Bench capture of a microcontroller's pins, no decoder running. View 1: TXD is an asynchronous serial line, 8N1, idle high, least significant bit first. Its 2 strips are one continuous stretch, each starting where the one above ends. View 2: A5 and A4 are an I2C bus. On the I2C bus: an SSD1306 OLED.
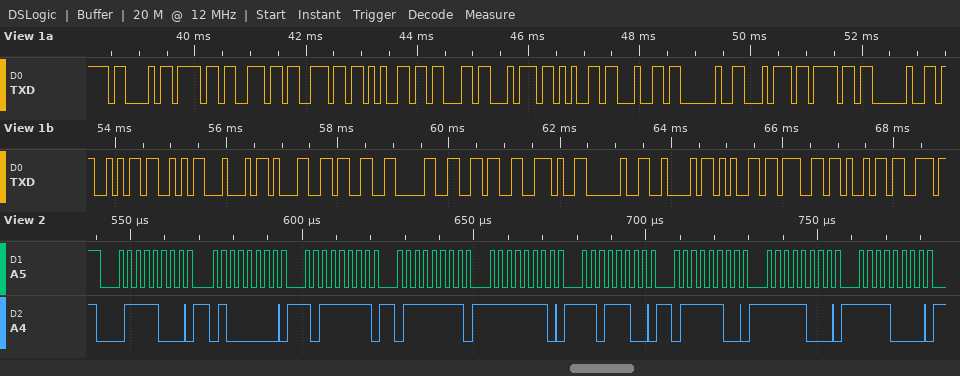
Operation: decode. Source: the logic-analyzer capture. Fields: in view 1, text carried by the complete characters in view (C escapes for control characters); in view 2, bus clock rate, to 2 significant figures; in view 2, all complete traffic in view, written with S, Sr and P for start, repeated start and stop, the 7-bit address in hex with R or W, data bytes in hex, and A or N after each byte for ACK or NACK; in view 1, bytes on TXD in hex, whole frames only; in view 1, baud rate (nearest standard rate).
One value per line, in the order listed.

"Connected to SSD1306. Begi"
400 kHz
S 3CW A 40 A BF A 7F A FE A DC A 7C A F8 A F0 A
43 6F 6E 6E 65 63 74 65 64 20 74 6F 20 53 53 44 31 33 30 36 2E 20 42 65 67 69
9600 baud
